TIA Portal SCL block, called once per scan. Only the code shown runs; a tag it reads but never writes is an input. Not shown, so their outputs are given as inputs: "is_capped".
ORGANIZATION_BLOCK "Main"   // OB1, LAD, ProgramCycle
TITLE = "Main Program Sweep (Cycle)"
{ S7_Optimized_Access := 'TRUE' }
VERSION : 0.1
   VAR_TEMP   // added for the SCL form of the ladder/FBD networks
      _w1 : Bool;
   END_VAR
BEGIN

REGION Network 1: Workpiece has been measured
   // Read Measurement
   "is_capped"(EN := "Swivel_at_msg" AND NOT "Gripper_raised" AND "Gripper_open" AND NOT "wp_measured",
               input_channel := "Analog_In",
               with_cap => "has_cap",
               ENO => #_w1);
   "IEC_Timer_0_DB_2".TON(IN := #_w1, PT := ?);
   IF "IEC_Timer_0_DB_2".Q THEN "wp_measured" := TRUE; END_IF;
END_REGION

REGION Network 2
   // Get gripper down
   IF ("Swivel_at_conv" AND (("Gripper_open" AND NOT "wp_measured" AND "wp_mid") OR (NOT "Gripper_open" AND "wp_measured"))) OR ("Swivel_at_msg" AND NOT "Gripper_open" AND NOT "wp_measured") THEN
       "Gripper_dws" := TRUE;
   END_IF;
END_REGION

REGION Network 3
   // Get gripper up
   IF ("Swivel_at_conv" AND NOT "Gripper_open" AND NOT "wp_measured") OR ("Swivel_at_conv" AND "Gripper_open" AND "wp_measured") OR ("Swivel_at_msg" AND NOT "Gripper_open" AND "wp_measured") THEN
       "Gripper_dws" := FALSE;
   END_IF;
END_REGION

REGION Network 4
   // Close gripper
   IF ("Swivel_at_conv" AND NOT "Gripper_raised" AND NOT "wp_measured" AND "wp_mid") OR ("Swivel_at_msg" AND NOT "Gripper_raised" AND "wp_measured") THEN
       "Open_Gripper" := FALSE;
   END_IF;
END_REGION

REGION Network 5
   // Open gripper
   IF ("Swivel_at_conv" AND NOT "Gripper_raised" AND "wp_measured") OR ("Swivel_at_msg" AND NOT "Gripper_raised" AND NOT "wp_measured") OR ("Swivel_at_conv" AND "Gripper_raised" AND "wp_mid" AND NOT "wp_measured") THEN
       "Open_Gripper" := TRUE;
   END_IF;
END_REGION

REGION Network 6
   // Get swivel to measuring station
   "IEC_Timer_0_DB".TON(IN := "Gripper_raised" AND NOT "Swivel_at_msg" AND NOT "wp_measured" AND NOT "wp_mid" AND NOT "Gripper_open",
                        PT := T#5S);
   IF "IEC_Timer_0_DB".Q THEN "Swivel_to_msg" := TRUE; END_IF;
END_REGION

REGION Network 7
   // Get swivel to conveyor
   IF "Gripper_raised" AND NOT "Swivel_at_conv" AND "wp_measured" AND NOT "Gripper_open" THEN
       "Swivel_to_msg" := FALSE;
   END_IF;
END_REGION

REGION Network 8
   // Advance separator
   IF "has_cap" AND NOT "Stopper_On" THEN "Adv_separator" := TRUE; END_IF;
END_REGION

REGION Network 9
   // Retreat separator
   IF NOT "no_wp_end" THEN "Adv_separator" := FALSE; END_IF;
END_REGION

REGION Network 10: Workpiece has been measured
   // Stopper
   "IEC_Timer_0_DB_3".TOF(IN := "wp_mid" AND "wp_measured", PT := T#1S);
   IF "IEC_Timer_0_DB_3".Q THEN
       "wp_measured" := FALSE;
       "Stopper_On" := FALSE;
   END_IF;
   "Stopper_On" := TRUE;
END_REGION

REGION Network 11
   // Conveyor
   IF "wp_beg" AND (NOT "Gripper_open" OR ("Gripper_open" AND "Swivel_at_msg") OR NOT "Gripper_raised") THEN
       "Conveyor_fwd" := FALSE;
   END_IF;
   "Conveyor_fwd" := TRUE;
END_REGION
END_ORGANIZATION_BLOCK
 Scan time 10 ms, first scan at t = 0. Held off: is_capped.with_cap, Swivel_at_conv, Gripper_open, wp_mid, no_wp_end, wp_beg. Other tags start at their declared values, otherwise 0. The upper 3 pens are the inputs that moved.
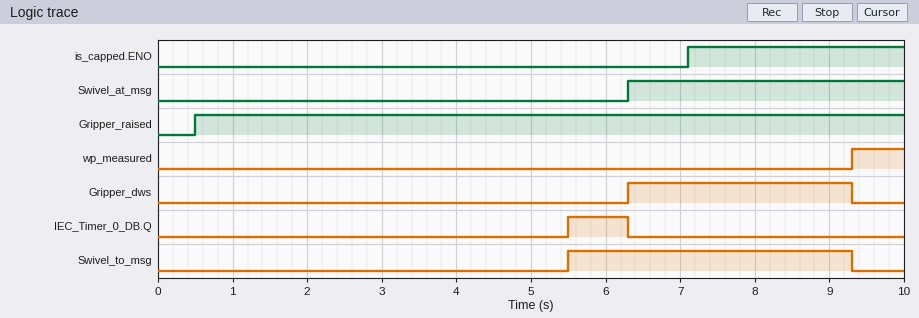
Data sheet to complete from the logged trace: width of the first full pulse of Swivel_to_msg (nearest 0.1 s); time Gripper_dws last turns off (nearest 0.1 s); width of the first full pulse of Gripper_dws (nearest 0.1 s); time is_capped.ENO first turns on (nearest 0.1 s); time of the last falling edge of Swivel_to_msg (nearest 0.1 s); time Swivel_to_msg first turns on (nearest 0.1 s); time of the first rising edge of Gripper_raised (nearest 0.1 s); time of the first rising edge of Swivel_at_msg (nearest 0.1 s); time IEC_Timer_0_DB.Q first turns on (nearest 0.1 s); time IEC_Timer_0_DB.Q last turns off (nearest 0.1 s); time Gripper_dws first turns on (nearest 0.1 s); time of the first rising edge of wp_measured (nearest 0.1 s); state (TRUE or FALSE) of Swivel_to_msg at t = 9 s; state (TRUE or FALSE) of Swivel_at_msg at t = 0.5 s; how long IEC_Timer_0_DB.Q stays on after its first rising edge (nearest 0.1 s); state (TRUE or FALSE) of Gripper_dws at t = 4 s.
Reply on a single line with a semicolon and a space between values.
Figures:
3.8 s; 9.3 s; 3.0 s; 7.1 s; 9.3 s; 5.5 s; 0.5 s; 6.3 s; 5.5 s; 6.3 s; 6.3 s; 9.3 s; TRUE; FALSE; 0.8 s; FALSE
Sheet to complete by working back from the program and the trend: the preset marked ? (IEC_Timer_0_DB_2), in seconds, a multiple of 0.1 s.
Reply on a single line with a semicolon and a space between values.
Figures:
2.2 s
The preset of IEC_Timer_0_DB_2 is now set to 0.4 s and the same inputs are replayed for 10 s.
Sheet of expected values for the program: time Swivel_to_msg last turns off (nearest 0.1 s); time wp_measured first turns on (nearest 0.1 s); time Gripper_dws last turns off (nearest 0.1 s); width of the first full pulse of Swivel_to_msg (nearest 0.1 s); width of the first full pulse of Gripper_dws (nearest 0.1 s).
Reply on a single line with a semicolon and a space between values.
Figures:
7.5 s; 7.5 s; 7.5 s; 2.0 s; 1.2 s
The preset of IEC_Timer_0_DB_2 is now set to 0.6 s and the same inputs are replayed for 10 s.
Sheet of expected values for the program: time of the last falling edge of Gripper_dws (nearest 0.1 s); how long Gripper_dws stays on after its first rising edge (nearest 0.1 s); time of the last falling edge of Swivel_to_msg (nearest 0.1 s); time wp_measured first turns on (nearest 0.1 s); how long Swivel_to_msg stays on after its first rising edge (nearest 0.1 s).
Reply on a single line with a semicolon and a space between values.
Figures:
7.7 s; 1.4 s; 7.7 s; 7.7 s; 2.2 s
